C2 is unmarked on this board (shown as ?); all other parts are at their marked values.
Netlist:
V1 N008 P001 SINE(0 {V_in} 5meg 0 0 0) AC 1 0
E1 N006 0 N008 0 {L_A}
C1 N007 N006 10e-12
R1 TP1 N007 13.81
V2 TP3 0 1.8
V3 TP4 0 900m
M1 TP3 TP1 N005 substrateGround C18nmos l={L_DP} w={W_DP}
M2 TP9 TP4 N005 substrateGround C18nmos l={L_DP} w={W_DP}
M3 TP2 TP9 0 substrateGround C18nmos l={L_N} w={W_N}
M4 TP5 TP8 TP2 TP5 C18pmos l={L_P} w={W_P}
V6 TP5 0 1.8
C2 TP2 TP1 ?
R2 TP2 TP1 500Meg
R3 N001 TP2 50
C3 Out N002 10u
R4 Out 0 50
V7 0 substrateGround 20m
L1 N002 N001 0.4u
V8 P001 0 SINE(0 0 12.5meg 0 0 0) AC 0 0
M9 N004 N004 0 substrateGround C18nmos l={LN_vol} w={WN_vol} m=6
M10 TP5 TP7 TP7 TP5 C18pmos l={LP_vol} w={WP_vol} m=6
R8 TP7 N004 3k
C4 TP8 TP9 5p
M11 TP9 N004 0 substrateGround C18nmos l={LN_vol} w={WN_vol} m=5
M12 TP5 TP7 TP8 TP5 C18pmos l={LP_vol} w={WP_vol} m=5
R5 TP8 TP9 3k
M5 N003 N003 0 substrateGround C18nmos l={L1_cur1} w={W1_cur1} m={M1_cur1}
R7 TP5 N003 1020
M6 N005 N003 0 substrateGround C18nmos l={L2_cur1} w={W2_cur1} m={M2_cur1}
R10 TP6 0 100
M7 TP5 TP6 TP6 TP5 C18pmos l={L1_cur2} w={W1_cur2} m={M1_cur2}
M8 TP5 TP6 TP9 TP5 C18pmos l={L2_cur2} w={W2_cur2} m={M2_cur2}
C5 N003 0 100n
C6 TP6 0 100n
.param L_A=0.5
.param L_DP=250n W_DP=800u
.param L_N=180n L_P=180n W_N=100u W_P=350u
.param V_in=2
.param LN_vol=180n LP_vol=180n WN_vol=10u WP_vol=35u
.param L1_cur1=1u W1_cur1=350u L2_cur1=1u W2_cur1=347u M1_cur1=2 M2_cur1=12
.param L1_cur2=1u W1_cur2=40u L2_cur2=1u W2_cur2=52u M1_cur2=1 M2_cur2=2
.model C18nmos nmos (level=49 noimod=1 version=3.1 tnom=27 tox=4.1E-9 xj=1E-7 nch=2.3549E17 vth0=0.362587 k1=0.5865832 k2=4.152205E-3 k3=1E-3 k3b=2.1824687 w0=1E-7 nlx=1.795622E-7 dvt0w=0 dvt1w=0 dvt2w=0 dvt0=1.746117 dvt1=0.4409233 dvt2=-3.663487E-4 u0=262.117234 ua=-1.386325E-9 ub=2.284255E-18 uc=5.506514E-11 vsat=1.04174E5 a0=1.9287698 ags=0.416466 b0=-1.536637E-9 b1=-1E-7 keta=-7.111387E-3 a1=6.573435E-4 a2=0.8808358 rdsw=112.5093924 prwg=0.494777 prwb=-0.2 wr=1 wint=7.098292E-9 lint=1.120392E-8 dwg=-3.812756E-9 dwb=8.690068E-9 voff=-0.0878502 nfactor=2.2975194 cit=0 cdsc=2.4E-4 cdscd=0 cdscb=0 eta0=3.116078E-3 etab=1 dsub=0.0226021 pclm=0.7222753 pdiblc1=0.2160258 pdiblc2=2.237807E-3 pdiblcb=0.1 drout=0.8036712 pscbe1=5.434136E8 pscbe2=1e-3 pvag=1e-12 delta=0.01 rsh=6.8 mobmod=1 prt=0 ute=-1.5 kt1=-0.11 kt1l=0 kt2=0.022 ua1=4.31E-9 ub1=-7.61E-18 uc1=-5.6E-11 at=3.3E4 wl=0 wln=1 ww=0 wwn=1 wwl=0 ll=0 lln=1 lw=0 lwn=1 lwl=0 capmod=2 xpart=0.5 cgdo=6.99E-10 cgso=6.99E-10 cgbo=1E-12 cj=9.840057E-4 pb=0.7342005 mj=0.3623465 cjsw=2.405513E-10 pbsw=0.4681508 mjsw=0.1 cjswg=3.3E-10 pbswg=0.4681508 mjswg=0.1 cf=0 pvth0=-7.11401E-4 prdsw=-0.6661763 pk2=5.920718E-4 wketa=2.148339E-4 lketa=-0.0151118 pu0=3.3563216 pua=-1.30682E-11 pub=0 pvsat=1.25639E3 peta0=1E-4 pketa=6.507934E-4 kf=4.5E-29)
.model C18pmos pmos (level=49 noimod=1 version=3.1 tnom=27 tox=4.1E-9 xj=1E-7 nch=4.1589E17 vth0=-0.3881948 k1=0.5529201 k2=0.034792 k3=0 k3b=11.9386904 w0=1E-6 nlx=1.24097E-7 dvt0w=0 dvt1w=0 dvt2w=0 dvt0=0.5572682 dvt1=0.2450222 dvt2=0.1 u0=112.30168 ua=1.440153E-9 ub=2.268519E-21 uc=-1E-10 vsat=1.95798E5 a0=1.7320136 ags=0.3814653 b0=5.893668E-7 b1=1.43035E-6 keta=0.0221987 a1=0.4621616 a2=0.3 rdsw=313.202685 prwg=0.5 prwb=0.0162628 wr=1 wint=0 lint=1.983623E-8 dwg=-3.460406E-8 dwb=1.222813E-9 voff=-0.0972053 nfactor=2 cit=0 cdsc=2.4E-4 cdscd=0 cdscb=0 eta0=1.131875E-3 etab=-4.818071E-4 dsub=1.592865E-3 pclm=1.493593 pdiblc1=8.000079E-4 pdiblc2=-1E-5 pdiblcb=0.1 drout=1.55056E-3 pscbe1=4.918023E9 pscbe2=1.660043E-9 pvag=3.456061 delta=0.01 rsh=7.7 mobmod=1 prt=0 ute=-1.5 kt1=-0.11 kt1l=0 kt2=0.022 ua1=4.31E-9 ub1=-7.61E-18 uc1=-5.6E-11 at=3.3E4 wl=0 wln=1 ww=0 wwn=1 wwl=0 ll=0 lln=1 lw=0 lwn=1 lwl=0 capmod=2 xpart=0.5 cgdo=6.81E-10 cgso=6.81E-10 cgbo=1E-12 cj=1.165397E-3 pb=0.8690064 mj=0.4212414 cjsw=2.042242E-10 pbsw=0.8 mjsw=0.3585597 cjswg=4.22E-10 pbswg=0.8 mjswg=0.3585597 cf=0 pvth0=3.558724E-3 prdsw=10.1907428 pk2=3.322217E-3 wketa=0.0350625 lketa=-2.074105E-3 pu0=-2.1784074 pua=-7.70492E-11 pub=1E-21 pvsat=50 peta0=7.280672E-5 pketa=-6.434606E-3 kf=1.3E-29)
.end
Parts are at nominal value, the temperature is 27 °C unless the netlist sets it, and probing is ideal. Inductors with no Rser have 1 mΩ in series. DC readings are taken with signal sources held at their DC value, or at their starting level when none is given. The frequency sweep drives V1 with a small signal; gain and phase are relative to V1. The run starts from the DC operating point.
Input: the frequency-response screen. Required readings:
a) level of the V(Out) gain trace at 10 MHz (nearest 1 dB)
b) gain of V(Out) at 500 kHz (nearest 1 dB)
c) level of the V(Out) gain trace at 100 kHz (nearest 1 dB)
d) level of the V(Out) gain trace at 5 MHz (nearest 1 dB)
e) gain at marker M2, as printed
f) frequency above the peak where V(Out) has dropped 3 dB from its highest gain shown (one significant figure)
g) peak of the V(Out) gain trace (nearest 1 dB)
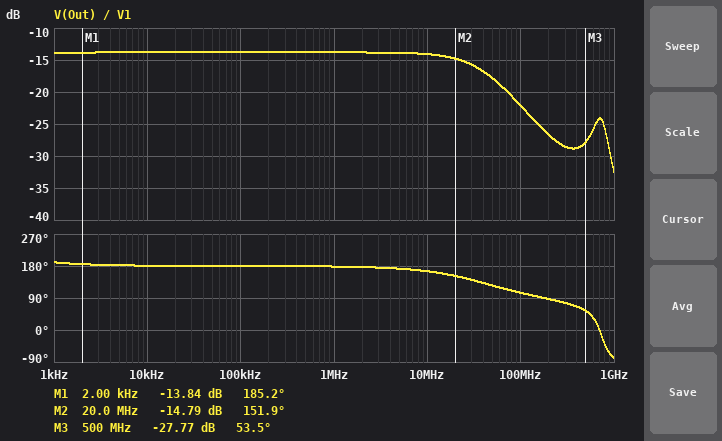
-14 dB
-14 dB
-14 dB
-14 dB
-14.79 dB
40 MHz
-14 dB
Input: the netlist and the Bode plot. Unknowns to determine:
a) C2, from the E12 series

12 pF
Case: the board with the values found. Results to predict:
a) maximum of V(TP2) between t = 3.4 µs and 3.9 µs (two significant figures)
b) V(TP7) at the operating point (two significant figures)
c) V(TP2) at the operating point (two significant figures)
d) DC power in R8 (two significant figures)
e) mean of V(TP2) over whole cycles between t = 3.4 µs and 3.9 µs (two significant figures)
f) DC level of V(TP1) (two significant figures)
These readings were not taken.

1.5 V
1.3 V
890 mV
170 µW
870 mV
890 mV
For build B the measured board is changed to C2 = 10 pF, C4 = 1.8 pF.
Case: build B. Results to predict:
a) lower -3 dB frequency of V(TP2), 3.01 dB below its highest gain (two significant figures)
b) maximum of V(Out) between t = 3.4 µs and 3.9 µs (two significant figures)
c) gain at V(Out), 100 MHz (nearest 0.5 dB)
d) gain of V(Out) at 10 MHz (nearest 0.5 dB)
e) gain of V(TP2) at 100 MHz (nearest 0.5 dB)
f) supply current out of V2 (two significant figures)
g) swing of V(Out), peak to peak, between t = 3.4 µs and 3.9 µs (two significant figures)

590 MHz
330 mV
-20.5 dB
-12.5 dB
-6.0 dB
3.7 mA
690 mV
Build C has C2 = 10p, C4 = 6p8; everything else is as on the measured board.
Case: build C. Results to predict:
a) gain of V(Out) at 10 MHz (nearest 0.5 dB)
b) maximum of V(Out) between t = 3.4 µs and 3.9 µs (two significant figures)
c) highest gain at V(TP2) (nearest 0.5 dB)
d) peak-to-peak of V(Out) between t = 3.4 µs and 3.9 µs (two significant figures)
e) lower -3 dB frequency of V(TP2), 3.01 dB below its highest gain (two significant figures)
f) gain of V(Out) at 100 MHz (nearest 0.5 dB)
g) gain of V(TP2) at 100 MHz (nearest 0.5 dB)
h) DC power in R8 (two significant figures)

-12.5 dB
330 mV
7.5 dB
690 mV
600 MHz
-20.5 dB
-6.0 dB
170 µW
